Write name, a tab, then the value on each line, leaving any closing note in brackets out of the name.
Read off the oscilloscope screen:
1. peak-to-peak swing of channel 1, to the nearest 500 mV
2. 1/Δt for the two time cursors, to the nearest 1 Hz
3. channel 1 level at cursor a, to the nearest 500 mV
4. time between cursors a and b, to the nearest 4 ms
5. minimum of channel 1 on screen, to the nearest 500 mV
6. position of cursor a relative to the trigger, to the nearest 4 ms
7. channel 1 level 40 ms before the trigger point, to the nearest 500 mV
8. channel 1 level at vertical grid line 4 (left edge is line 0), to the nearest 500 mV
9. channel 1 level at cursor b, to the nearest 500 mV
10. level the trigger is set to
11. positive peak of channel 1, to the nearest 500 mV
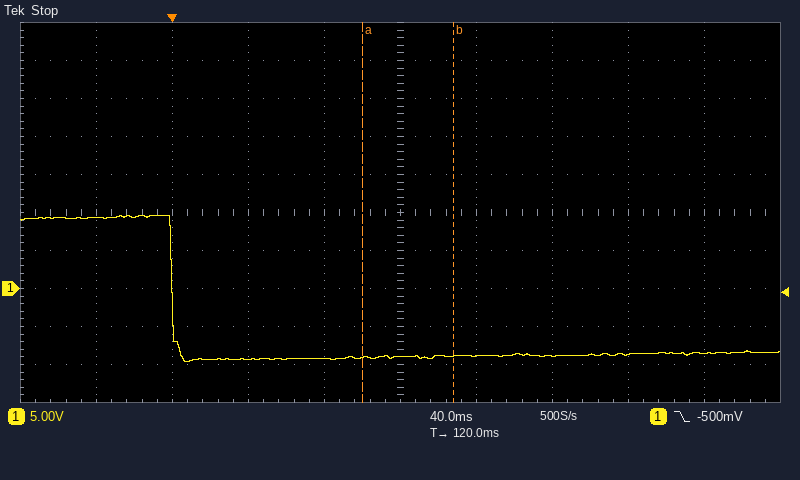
peak-to-peak swing of channel 1, to the nearest 500 mV	19.0 V
1/Δt for the two time cursors, to the nearest 1 Hz	21 Hz
channel 1 level at cursor a, to the nearest 500 mV	-9.0 V
time between cursors a and b, to the nearest 4 ms	48 ms
minimum of channel 1 on screen, to the nearest 500 mV	-9.5 V
position of cursor a relative to the trigger, to the nearest 4 ms	+100 ms
channel 1 level 40 ms before the trigger point, to the nearest 500 mV	9.5 V
channel 1 level at vertical grid line 4 (left edge is line 0), to the nearest 500 mV	-9.0 V
channel 1 level at cursor b, to the nearest 500 mV	-9.0 V
level the trigger is set to	-500 mV
positive peak of channel 1, to the nearest 500 mV	9.5 V
